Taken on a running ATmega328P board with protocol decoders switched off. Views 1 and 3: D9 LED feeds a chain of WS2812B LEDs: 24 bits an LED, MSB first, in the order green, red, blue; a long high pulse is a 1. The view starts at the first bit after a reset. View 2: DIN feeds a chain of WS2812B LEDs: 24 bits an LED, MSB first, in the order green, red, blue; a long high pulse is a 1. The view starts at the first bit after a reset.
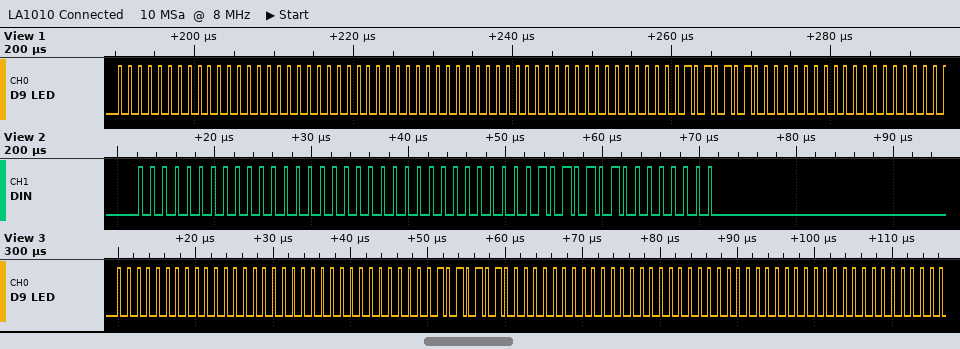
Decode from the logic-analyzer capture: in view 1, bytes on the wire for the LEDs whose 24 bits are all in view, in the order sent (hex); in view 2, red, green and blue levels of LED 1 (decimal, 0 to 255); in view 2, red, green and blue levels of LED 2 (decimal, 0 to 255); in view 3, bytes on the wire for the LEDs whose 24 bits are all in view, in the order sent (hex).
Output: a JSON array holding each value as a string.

["00 00 00 00 00 00 00 55 00", "0, 0, 0", "85, 0, 0", "00 00 00 00 55 00 00 00 00"]
